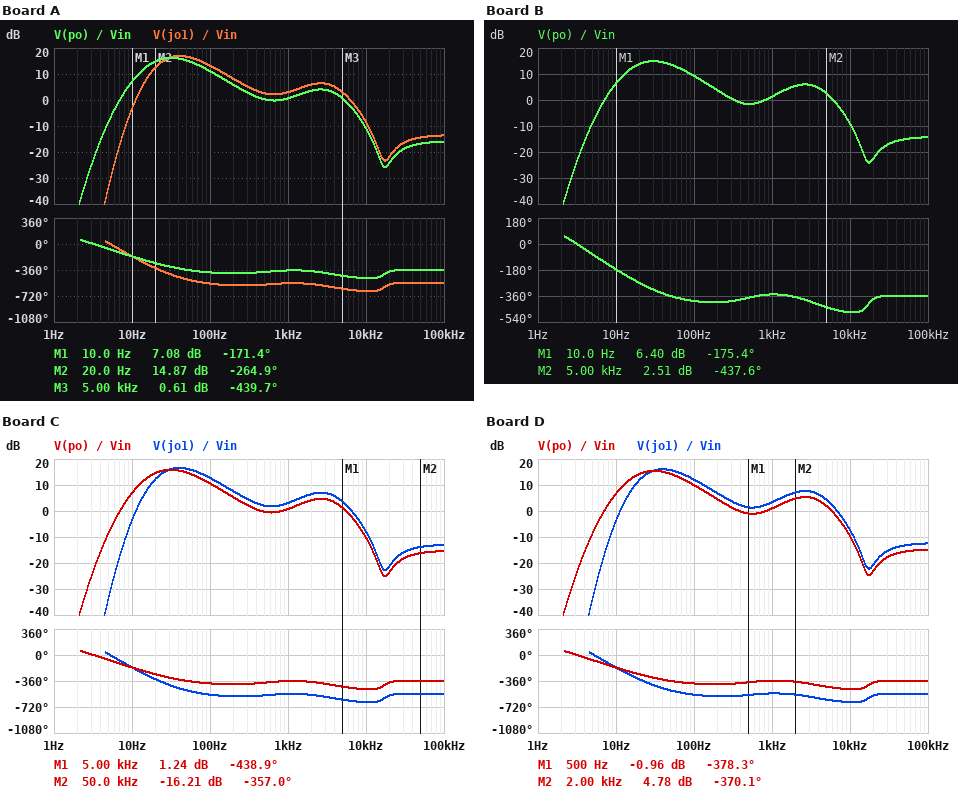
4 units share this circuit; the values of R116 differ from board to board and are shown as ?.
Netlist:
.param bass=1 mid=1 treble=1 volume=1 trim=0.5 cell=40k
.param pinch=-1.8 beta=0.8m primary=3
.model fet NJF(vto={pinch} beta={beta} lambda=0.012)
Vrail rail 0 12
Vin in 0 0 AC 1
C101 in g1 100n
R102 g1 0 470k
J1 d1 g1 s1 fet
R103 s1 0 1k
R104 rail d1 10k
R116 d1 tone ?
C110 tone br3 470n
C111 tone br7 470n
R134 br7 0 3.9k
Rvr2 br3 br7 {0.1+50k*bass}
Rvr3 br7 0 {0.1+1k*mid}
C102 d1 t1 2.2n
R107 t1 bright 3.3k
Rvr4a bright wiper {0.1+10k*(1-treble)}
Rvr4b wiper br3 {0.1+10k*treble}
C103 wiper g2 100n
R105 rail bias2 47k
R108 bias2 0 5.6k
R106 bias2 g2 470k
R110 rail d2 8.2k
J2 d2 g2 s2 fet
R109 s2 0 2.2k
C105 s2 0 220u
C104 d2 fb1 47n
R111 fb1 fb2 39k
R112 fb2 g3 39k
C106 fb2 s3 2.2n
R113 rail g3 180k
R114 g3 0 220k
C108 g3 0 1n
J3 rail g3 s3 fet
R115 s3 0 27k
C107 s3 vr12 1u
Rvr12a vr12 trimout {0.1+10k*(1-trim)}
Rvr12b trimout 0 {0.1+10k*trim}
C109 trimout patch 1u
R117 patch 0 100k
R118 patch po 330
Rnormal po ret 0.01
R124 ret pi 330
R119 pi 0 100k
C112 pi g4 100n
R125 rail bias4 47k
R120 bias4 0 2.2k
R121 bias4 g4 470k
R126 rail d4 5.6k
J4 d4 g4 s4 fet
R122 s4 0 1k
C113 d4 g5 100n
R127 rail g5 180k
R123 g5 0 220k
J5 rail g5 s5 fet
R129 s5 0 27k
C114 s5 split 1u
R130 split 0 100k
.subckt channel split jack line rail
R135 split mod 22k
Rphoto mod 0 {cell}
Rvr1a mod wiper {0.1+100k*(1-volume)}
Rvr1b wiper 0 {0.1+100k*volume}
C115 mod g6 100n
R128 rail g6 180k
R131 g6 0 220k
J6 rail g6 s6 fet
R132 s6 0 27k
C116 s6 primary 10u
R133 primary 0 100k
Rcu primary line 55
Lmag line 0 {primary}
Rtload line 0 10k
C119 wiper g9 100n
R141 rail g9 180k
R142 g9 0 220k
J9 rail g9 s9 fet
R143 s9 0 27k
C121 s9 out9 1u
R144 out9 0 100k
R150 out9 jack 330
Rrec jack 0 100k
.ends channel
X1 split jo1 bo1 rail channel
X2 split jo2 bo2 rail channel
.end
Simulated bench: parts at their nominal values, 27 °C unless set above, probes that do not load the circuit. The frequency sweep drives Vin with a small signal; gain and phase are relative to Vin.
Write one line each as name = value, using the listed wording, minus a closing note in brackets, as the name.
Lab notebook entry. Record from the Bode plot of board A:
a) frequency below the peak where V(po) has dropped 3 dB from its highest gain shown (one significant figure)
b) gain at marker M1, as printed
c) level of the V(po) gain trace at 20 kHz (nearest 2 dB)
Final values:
frequency below the peak where V(po) has dropped 3 dB from its highest gain shown = 20 Hz
gain at marker M1, as printed = 7.08 dB
level of the V(po) gain trace at 20 kHz = -24 dB
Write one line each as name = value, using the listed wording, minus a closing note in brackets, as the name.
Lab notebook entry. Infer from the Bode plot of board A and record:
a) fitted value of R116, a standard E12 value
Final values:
fitted value of R116, a standard E12 value = 4.7 kΩ
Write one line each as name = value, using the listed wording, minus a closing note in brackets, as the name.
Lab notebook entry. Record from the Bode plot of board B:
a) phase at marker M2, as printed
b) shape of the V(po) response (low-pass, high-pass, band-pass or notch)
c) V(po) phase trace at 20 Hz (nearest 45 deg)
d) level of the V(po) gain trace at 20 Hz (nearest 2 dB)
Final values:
phase at marker M2, as printed = -437.6 deg
shape of the V(po) response = band-pass
V(po) phase trace at 20 Hz = -270 deg
level of the V(po) gain trace at 20 Hz = 14 dB
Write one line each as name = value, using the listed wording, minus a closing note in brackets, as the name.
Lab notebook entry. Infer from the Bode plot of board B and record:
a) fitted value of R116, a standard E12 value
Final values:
fitted value of R116, a standard E12 value = 8.2 kΩ
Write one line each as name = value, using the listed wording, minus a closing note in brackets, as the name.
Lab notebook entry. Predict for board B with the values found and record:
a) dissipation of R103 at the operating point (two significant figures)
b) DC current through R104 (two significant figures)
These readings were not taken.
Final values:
dissipation of R103 at the operating point = 660 µW
DC current through R104 = 810 µA
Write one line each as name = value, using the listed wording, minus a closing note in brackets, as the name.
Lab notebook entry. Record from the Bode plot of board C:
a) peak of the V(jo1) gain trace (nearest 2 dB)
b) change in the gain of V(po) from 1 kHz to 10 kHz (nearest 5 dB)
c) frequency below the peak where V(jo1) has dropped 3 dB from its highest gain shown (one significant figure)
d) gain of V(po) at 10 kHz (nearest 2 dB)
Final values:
peak of the V(jo1) gain trace = 16 dB
change in the gain of V(po) from 1 kHz to 10 kHz = -10 dB
frequency below the peak where V(jo1) has dropped 3 dB from its highest gain shown = 20 Hz
gain of V(po) at 10 kHz = -10 dB
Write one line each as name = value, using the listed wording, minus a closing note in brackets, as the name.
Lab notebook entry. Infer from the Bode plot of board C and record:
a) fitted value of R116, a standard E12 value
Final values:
fitted value of R116, a standard E12 value = 5.6 kΩ
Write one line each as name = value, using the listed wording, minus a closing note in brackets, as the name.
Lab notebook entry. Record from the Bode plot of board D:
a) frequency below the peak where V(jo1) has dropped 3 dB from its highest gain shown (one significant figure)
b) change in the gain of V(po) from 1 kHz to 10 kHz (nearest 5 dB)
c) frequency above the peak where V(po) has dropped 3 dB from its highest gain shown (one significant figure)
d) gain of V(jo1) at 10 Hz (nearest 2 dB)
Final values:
frequency below the peak where V(jo1) has dropped 3 dB from its highest gain shown = 20 Hz
change in the gain of V(po) from 1 kHz to 10 kHz = -10 dB
frequency above the peak where V(po) has dropped 3 dB from its highest gain shown = 70 Hz
gain of V(jo1) at 10 Hz = -4 dB
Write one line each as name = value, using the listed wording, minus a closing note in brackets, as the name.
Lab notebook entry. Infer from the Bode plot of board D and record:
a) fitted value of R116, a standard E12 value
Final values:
fitted value of R116, a standard E12 value = 6.8 kΩ
